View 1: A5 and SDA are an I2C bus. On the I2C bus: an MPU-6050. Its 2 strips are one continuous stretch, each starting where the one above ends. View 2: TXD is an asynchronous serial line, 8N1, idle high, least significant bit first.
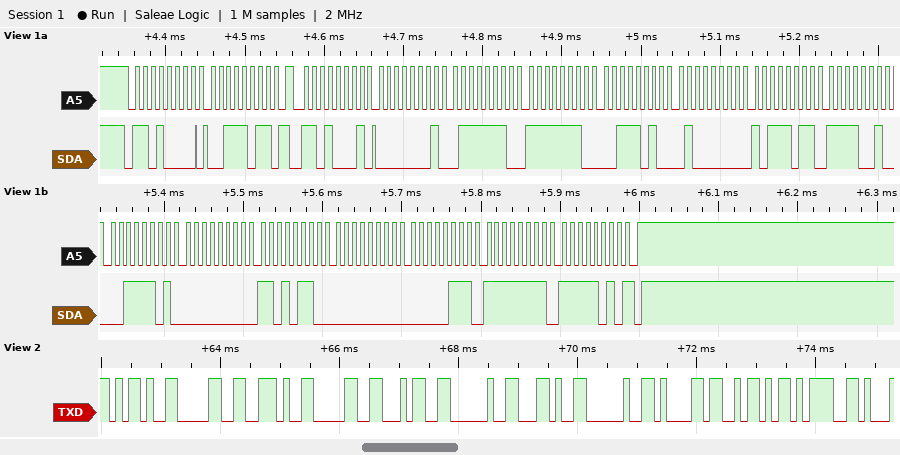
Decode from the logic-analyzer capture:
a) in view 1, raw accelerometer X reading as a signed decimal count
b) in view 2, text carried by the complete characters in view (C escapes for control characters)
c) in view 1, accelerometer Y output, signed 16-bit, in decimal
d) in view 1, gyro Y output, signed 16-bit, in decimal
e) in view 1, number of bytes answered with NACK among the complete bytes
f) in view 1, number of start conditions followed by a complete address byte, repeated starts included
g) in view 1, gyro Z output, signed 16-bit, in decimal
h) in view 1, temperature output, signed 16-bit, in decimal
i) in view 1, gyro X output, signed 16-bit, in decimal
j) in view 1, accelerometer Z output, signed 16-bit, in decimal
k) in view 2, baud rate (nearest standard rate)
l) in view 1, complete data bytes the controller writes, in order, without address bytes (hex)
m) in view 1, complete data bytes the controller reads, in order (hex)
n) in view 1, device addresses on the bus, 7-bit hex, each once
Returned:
382
"-0.04 , aZ="
-454
7
1
2
-6
-3523
214
16571
9600 baud
3B
01 7E FE 3A 40 BB F2 3D 00 D6 00 07 FF FA
0x68
